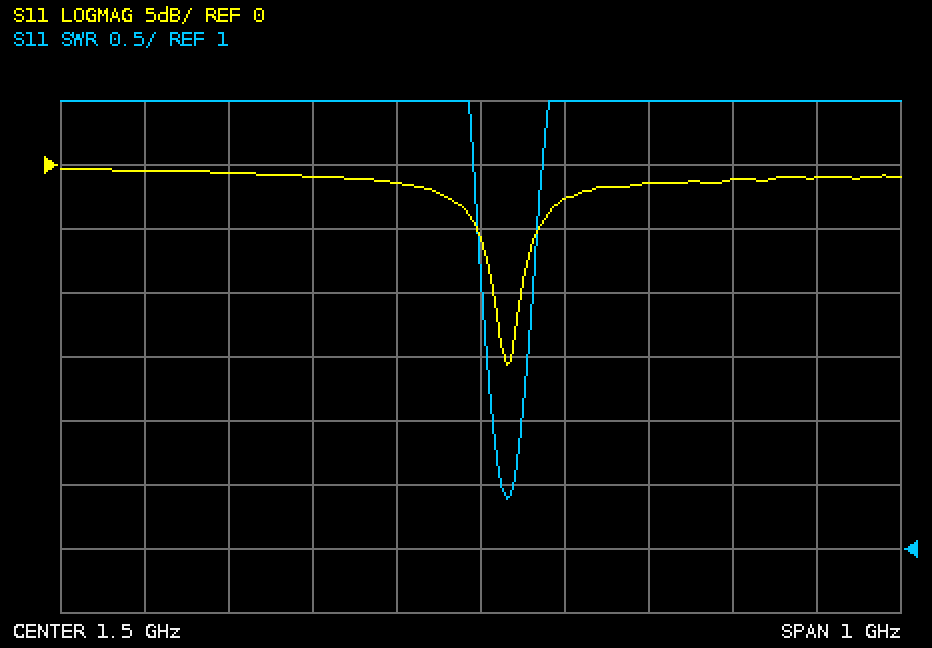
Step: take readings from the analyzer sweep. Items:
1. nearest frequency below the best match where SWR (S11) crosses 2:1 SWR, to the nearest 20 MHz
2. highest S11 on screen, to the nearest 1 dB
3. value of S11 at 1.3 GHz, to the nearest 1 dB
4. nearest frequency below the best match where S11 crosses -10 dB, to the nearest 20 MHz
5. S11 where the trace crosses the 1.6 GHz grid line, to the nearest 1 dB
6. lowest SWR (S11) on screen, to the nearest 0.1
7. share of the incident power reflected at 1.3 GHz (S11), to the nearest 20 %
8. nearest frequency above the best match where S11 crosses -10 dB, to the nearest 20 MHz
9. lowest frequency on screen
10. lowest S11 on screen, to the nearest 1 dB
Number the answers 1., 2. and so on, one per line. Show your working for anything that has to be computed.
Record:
1. 1.52 GHz
2. 0 dB
3. -1 dB
4. 1.52 GHz
5. -3 dB
6. 1.4
7. 10^(-1/10) ≈ 79.4 %, so 80 % to the nearest 20 %
8. 1.54 GHz
9. 1 GHz
10. -16 dB
